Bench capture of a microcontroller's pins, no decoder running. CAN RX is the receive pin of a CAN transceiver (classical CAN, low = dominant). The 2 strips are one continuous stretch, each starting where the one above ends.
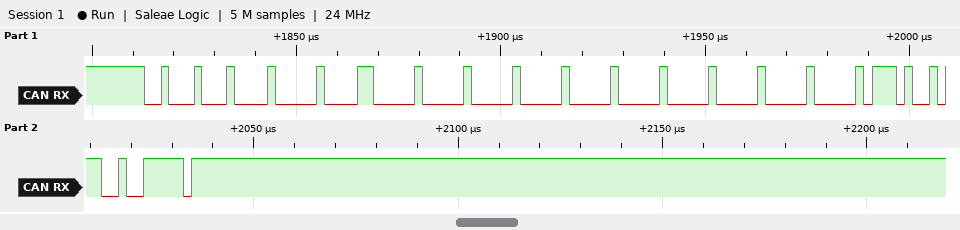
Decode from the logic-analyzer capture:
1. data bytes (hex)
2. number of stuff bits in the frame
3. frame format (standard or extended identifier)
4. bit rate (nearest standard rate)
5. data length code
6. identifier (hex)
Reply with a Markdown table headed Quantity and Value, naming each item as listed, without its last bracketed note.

| Quantity | Value |
|---|---|
| data bytes | 03 00 00 00 00 00 00 1D |
| number of stuff bits in the frame | 11 |
| frame format | standard |
| bit rate | 500 kbit/s |
| data length code | 8 |
| identifier | 0x222 |
